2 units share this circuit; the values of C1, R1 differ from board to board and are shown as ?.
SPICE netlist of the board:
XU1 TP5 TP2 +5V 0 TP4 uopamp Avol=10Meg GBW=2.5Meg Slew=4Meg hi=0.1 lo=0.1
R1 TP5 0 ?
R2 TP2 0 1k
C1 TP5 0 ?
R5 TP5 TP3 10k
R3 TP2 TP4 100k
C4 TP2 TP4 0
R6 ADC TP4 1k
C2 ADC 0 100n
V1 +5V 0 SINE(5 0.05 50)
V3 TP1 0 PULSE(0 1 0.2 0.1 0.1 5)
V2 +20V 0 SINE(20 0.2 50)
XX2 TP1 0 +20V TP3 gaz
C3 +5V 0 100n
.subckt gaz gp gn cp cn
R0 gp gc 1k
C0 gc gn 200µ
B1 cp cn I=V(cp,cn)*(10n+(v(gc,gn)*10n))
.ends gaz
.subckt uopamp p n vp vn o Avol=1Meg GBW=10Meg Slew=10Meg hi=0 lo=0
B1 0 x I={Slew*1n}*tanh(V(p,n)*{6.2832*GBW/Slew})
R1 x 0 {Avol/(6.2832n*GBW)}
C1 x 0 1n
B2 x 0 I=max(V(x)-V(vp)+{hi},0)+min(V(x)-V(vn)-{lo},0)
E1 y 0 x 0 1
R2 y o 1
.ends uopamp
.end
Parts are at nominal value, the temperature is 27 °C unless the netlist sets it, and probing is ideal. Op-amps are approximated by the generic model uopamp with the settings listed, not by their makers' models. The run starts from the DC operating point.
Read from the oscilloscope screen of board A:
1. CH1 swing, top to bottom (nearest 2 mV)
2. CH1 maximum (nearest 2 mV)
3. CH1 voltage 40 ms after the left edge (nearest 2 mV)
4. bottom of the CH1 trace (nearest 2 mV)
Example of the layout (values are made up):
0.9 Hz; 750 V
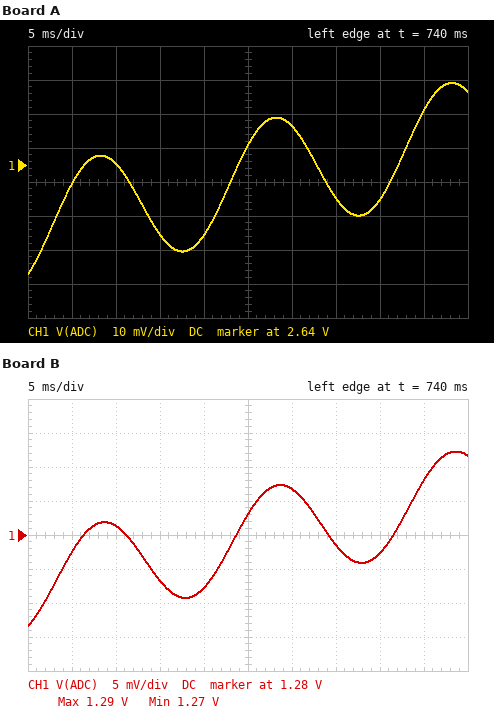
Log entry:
56 mV; 2.664 V; 2.630 V; 2.608 V
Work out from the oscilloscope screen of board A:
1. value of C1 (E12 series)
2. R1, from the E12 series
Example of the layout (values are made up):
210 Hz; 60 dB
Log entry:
56 nF; 68 kΩ
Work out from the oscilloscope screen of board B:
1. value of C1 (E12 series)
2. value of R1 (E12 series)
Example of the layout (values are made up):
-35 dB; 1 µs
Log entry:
150 nF; 33 kΩ
